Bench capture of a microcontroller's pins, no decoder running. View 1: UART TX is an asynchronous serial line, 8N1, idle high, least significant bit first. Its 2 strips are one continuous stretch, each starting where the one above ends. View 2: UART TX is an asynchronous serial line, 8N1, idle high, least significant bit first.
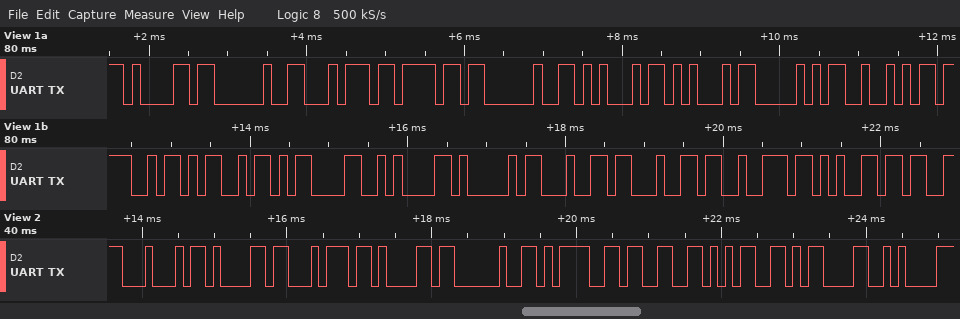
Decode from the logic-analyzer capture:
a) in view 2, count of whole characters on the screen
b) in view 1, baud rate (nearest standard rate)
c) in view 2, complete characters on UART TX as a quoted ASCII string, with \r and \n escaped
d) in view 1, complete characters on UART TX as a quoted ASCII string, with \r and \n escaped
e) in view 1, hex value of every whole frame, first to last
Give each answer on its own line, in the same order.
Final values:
10
9600 baud
"Data =35\r\n"
"a to EEPROM\r\nAddre"
0x61 0x20 0x74 0x6F 0x20 0x45 0x45 0x50 0x52 0x4F 0x4D 0x0D 0x0A 0x41 0x64 0x64 0x72 0x65
